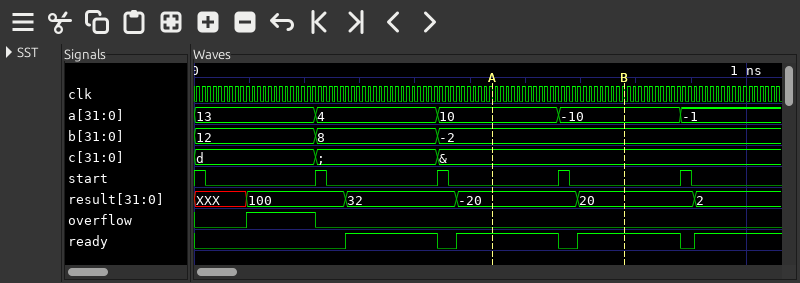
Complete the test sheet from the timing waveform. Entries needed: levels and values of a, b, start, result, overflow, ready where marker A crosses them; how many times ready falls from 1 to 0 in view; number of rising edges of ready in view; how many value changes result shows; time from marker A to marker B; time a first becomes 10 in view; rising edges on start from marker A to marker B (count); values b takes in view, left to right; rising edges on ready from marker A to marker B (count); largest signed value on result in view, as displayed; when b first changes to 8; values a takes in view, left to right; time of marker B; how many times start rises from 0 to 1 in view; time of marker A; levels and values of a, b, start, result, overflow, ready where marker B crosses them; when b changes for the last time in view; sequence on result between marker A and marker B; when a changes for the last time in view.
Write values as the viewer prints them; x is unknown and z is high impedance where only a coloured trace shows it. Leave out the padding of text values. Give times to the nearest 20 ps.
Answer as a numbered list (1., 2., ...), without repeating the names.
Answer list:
1. a=10, b=-2, start=0, result=-20, overflow=0, ready=1
2. 3
3. 4
4. 5
5. 240 ps
6. 440 ps
7. 1
8. 12, 8, -2
9. 1
10. 100
11. 220 ps
12. 13, 4, 10, -10, -1
13. 780 ps
14. 4
15. 540 ps
16. a=-10, b=-2, start=0, result=20, overflow=0, ready=1
17. 440 ps
18. -20, 20
19. 880 ps
